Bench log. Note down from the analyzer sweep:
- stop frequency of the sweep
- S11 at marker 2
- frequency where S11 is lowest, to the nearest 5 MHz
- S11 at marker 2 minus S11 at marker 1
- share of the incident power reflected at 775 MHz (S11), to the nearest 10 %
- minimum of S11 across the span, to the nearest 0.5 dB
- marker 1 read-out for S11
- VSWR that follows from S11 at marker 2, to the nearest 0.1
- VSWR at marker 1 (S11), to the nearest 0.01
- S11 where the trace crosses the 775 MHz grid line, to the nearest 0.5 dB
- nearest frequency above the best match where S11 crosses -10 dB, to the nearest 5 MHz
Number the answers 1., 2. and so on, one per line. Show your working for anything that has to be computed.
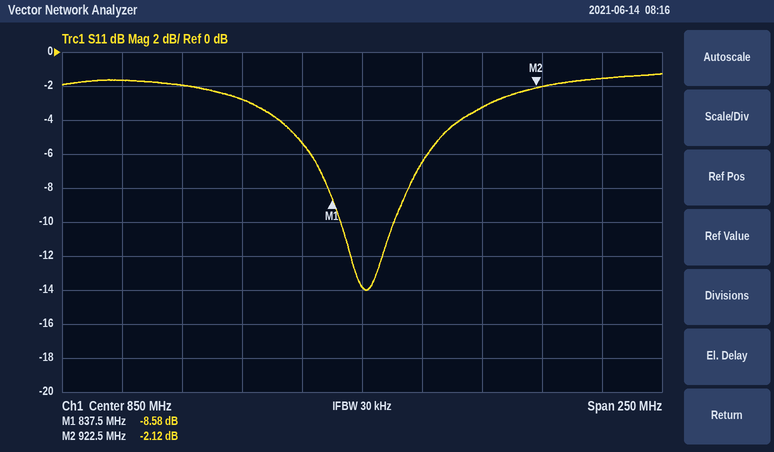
1. 975 MHz
2. -2.12 dB
3. 850 MHz
4. -2.12 − (-8.58) = 6.46 dB
5. 10^(-2/10) ≈ 63.1 %, so 60 % to the nearest 10 %
6. -14.0 dB
7. -8.58 dB
8. (1 + 0.7834)/(1 − 0.7834) ≈ 8.2
9. (1 + 0.3724)/(1 − 0.3724) ≈ 2.19
10. -2.0 dB
11. 865 MHz
